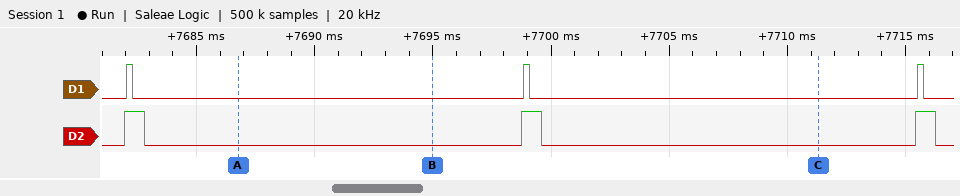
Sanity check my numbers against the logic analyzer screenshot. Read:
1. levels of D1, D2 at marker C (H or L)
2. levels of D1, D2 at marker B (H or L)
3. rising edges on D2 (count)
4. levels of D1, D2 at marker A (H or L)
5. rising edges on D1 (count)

D1=L, D2=L
D1=L, D2=L
3
D1=L, D2=L
3
